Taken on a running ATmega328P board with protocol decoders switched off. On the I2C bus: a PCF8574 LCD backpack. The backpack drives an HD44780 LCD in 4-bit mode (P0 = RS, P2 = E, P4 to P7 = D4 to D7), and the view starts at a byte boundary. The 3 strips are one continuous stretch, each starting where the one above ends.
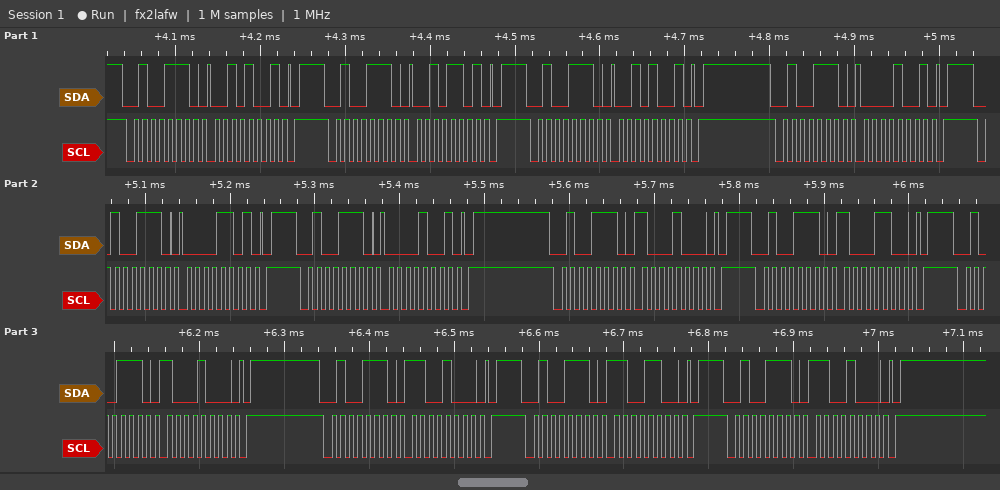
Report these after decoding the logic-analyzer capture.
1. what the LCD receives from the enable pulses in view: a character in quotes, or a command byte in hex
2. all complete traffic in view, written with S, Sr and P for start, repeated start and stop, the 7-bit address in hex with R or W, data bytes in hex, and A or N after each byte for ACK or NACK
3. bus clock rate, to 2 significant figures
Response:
' ' 0x8C
S 27W A 29 A P S 27W A 2D A P S 27W A 29 A P S 27W A 09 A P S 27W A 0D A P S 27W A 09 A P S 27W A 88 A P S 27W A 8C A P S 27W A 88 A P S 27W A C8 A P S 27W A CC A P S 27W A C8 A P
100 kHz
